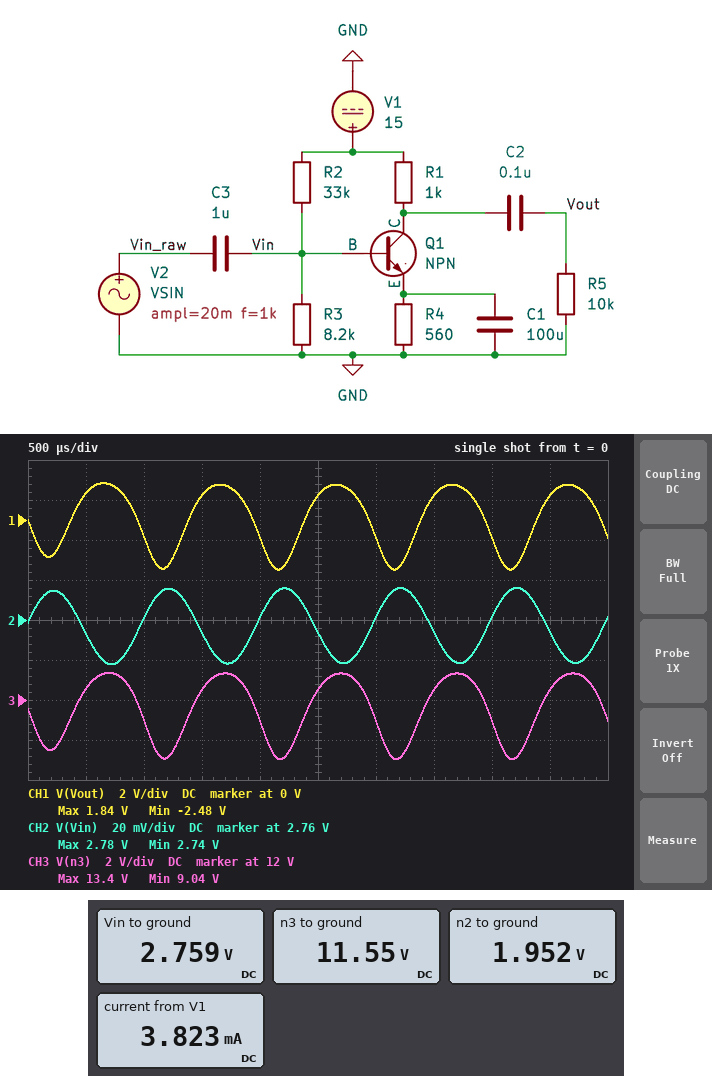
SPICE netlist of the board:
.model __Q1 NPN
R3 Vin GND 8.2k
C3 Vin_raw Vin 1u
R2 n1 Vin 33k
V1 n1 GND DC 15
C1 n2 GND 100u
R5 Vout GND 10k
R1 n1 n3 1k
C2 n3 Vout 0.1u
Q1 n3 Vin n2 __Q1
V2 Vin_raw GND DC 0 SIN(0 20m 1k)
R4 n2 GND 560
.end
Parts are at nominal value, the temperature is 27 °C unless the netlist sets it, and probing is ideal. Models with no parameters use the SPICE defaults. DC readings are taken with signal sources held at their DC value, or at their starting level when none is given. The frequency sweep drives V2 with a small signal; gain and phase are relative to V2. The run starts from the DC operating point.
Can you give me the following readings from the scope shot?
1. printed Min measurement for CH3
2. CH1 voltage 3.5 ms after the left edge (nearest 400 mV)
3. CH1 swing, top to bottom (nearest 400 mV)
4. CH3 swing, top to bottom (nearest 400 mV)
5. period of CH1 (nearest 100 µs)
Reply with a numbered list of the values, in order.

1. 9.04 V
2. 1.2 V
3. 4.4 V
4. 4.4 V
5. 1.0 ms
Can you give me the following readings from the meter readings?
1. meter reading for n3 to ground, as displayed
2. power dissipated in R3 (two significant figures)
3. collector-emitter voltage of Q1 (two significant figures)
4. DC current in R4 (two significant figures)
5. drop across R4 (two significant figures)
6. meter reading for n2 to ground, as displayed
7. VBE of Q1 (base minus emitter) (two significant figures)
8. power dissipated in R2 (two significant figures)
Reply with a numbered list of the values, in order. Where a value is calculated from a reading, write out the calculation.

1. 11.55 V
2. (2.759 V)^2 / 8.2 kΩ = 930 µW
3. 11.55 V - 1.952 V = 9.6 V
4. (1.952 V) / 560 Ω = 3.5 mA
5. 1.952 V = 2.0 V
6. 1.952 V
7. 2.759 V - 1.952 V = 810 mV
8. (15 V - 2.759 V)^2 / 33 kΩ = 4.5 mW
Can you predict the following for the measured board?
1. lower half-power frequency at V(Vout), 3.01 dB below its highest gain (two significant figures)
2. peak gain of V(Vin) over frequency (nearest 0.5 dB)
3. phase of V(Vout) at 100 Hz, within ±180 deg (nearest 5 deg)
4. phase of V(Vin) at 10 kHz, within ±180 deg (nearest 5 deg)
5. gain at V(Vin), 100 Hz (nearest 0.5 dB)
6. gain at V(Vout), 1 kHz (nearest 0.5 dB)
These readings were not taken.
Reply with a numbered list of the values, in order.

1. 480 Hz
2. 0 dB
3. -40 deg
4. 0 deg
5. -5.5 dB
6. 41.0 dB
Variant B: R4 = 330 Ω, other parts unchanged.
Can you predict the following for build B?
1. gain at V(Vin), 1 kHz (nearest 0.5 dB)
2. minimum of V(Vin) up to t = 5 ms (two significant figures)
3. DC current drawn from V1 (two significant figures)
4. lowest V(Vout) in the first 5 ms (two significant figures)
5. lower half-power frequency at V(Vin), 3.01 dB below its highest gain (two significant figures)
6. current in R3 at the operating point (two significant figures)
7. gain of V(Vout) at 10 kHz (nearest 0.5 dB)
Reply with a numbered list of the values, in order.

1. -1.0 dB
2. 2.6 V
3. 5.8 mA
4. -3.5 V
5. 490 Hz
6. 320 µA
7. 45.5 dB
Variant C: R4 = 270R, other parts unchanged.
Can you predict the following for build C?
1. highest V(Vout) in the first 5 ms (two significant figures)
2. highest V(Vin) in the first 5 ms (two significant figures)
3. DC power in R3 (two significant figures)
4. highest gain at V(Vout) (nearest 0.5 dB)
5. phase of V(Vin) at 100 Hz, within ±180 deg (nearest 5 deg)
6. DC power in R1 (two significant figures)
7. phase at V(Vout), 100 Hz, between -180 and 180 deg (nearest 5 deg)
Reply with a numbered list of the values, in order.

1. 2.9 V
2. 2.6 V
3. 800 µW
4. 47.0 dB
5. 15 deg
6. 41 mW
7. -35 deg
